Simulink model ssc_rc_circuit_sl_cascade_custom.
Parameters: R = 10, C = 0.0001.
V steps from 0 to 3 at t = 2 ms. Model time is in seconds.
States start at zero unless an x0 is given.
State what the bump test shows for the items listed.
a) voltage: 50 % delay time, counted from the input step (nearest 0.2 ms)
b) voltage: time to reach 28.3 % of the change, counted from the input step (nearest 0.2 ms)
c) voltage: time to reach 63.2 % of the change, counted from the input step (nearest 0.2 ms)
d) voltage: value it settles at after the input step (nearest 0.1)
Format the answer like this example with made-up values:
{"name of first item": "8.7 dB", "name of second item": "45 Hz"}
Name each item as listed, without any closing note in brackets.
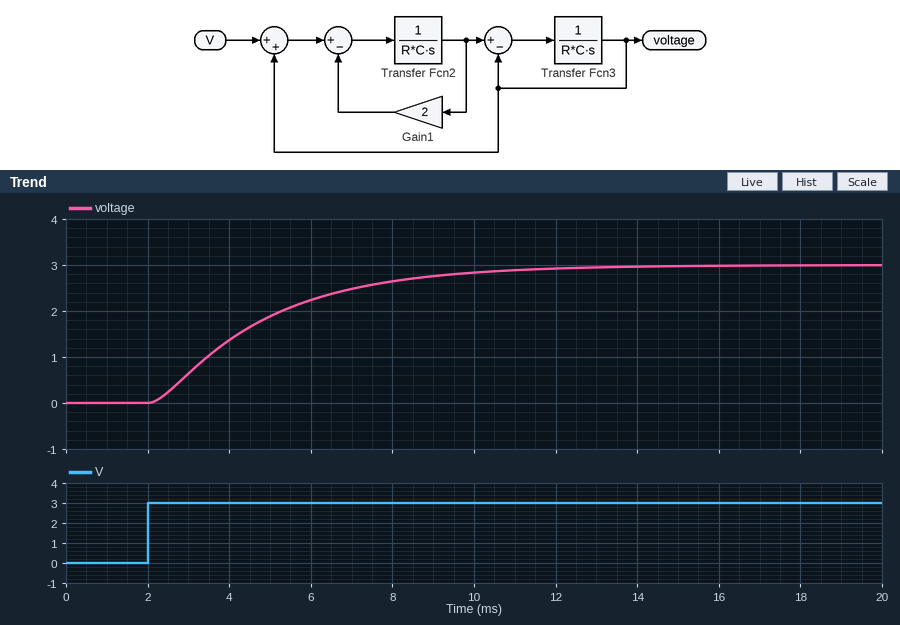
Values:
{"voltage: 50 % delay time, counted from the input step": "2.2 ms", "voltage: time to reach 28.3 % of the change, counted from the input step": "1.2 ms", "voltage: time to reach 63.2 % of the change, counted from the input step": "3.0 ms", "voltage: value it settles at after the input step": "3.0"}
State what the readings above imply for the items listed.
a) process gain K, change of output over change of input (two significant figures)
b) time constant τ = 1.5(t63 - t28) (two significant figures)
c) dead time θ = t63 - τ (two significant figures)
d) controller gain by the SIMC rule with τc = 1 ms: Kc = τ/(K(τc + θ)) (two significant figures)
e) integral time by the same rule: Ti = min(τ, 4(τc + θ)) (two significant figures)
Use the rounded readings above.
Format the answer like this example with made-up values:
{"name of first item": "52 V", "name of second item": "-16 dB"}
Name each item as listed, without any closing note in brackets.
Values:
{"process gain K, change of output over change of input": "1.0", "time constant τ = 1.5(t63 - t28)": "2.7 ms", "dead time θ = t63 - τ": "0.30 ms", "controller gain by the SIMC rule with τc = 1 ms: Kc = τ/(K(τc + θ))": "2.1", "integral time by the same rule: Ti = min(τ, 4(τc + θ))": "2.7 ms"}
